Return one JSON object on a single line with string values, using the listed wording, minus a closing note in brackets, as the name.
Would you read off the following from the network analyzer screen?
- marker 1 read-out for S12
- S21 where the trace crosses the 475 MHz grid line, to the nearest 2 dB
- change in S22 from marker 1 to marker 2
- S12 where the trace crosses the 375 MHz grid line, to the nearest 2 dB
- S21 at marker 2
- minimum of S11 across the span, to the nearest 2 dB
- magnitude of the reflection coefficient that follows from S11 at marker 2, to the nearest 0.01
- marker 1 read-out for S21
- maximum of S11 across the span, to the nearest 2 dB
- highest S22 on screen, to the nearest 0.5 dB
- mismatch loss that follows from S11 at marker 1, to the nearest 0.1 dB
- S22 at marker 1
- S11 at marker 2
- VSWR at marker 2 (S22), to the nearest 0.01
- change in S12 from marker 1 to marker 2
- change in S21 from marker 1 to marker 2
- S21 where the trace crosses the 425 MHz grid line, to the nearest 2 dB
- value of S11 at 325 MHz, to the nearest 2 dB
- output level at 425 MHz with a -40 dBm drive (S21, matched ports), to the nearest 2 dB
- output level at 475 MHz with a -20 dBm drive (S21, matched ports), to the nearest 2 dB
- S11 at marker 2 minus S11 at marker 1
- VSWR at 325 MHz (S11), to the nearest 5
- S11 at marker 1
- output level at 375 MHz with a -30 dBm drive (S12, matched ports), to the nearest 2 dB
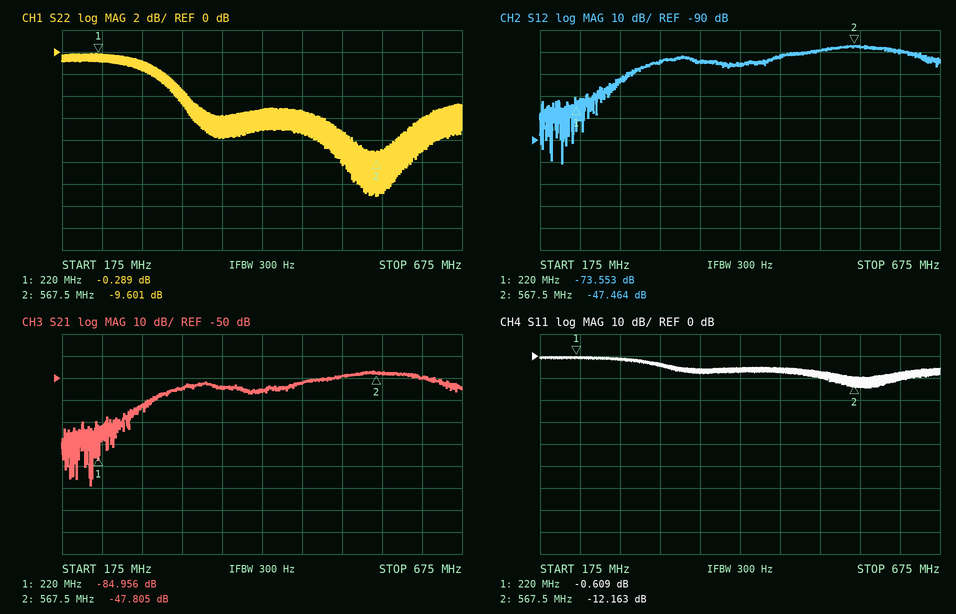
{"marker 1 read-out for S12": "-73.553 dB", "S21 where the trace crosses the 475 MHz grid line, to the nearest 2 dB": "-52 dB", "change in S22 from marker 1 to marker 2": "-9.312 dB", "S12 where the trace crosses the 375 MHz grid line, to the nearest 2 dB": "-54 dB", "S21 at marker 2": "-47.805 dB", "minimum of S11 across the span, to the nearest 2 dB": "-14 dB", "magnitude of the reflection coefficient that follows from S11 at marker 2, to the nearest 0.01": "0.25", "marker 1 read-out for S21": "-84.956 dB", "maximum of S11 across the span, to the nearest 2 dB": "0 dB", "highest S22 on screen, to the nearest 0.5 dB": "0.0 dB", "mismatch loss that follows from S11 at marker 1, to the nearest 0.1 dB": "8.8 dB", "S22 at marker 1": "-0.289 dB", "S11 at marker 2": "-12.163 dB", "VSWR at marker 2 (S22), to the nearest 0.01": "1.99", "change in S12 from marker 1 to marker 2": "26.089 dB", "change in S21 from marker 1 to marker 2": "37.151 dB", "S21 where the trace crosses the 425 MHz grid line, to the nearest 2 dB": "-56 dB", "value of S11 at 325 MHz, to the nearest 2 dB": "-4 dB", "output level at 425 MHz with a -40 dBm drive (S21, matched ports), to the nearest 2 dB": "-96 dBm", "output level at 475 MHz with a -20 dBm drive (S21, matched ports), to the nearest 2 dB": "-72 dBm", "S11 at marker 2 minus S11 at marker 1": "-11.554 dB", "VSWR at 325 MHz (S11), to the nearest 5": "5", "S11 at marker 1": "-0.609 dB", "output level at 375 MHz with a -30 dBm drive (S12, matched ports), to the nearest 2 dB": "-84 dBm"}
